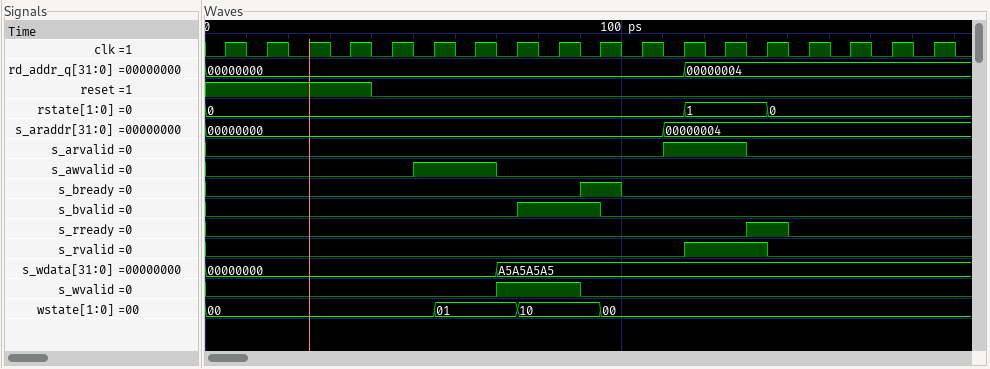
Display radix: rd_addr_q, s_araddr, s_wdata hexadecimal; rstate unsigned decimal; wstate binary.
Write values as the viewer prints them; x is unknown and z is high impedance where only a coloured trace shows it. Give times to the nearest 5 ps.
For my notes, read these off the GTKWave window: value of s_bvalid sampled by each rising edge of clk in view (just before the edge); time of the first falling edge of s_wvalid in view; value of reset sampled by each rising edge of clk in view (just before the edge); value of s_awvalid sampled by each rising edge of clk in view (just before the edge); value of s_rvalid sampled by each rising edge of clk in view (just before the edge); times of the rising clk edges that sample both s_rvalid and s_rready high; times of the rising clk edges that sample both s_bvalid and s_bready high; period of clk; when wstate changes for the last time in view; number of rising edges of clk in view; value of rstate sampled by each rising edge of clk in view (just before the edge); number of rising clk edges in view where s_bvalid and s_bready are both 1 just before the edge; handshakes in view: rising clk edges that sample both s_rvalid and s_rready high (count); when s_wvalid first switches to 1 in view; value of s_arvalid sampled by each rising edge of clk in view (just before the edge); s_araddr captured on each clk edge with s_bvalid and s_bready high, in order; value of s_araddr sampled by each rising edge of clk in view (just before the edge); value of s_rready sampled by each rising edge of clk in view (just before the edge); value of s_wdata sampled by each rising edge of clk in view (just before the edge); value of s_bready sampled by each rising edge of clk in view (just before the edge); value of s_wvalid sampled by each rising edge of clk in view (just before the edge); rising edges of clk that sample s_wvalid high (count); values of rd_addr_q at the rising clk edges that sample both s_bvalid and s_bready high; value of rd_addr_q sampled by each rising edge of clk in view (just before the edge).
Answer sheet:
0 0 0 0 0 0 0 0 1 1 0 0 0 0 0 0 0 0
90 ps
1 1 1 1 0 0 0 0 0 0 0 0 0 0 0 0 0 0
0 0 0 0 0 1 1 0 0 0 0 0 0 0 0 0 0 0
0 0 0 0 0 0 0 0 0 0 0 0 1 1 0 0 0 0
135 ps
95 ps
10 ps
95 ps
18
0, 0, 0, 0, 0, 0, 0, 0, 0, 0, 0, 0, 1, 1, 0, 0, 0, 0
1
1
70 ps
0 0 0 0 0 0 0 0 0 0 0 1 1 0 0 0 0 0
00000000
00000000, 00000000, 00000000, 00000000, 00000000, 00000000, 00000000, 00000000, 00000000, 00000000, 00000000, 00000004, 00000004, 00000004, 00000004, 00000004, 00000004, 00000004
0 0 0 0 0 0 0 0 0 0 0 0 0 1 0 0 0 0
00000000, 00000000, 00000000, 00000000, 00000000, 00000000, 00000000, A5A5A5A5, A5A5A5A5, A5A5A5A5, A5A5A5A5, A5A5A5A5, A5A5A5A5, A5A5A5A5, A5A5A5A5, A5A5A5A5, A5A5A5A5, A5A5A5A5
0 0 0 0 0 0 0 0 0 1 0 0 0 0 0 0 0 0
0 0 0 0 0 0 0 1 1 0 0 0 0 0 0 0 0 0
2
00000000
00000000, 00000000, 00000000, 00000000, 00000000, 00000000, 00000000, 00000000, 00000000, 00000000, 00000000, 00000000, 00000004, 00000004, 00000004, 00000004, 00000004, 00000004
